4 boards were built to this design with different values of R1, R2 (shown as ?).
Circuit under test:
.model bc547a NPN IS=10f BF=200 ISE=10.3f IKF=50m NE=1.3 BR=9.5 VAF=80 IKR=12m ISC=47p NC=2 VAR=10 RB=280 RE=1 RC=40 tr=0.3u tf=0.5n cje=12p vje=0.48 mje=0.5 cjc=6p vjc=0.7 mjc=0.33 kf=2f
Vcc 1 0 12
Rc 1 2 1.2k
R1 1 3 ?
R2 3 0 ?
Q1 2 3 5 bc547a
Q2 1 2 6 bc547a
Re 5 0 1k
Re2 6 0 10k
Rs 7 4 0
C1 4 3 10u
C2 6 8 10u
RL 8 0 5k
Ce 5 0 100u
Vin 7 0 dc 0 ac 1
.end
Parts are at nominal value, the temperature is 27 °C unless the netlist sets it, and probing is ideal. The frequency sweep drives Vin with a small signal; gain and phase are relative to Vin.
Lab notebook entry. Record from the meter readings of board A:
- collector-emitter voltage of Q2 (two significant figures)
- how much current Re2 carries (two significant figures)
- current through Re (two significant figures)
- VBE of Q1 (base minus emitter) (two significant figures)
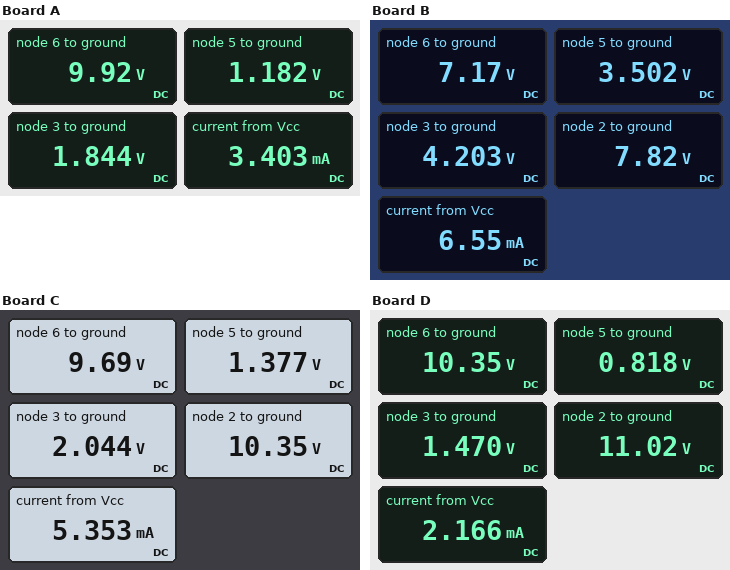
2.1 V
990 µA
1.2 mA
660 mV
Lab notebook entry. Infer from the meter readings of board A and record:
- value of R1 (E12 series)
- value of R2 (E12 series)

8.2 kΩ
1.5 kΩ
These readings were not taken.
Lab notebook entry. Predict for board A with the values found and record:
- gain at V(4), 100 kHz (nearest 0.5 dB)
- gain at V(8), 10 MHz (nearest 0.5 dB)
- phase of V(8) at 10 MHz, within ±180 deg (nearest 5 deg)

0 dB
22.0 dB
95 deg
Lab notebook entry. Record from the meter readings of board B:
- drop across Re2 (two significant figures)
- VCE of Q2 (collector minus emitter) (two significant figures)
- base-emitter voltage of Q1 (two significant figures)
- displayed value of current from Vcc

7.2 V
4.8 V
700 mV
6.55 mA
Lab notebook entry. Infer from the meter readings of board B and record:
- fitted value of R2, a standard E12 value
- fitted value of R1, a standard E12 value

1.8 kΩ
3.3 kΩ
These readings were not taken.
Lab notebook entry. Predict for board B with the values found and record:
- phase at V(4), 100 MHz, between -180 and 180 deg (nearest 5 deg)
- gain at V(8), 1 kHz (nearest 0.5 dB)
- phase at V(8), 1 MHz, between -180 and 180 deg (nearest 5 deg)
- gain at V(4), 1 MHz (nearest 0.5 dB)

0 deg
40.0 dB
140 deg
0 dB
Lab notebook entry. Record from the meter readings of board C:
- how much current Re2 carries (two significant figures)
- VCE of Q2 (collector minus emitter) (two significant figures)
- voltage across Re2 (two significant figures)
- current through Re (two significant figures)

970 µA
2.3 V
9.7 V
1.4 mA
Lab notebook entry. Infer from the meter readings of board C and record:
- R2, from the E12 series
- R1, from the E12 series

680 Ω
3.3 kΩ
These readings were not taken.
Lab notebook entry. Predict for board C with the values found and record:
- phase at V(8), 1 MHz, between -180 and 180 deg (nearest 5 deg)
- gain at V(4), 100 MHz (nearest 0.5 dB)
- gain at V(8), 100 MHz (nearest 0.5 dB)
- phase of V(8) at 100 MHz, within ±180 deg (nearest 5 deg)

160 deg
0 dB
-4.0 dB
20 deg
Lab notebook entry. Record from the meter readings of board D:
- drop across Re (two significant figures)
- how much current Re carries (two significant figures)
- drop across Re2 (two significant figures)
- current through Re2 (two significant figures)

820 mV
820 µA
10 V
1.0 mA
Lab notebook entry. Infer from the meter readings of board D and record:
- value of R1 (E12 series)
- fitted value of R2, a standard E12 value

33 kΩ
4.7 kΩ
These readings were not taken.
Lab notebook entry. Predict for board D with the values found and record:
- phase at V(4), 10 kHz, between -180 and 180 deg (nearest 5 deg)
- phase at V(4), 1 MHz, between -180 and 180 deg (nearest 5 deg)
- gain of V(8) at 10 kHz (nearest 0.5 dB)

0 deg
0 deg
30.5 dB
